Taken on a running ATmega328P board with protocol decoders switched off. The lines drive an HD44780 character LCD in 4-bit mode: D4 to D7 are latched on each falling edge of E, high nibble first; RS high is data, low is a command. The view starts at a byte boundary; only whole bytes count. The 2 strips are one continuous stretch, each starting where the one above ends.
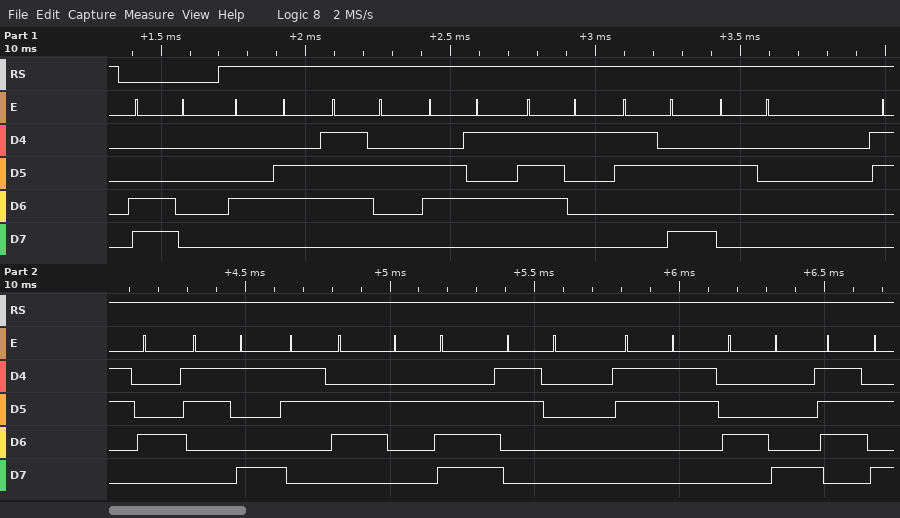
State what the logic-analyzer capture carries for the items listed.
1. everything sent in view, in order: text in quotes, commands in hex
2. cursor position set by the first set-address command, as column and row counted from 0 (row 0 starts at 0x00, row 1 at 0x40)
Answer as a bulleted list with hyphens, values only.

- 0xC0 "Freq: 496.03Hz"
- column 0, row 1
